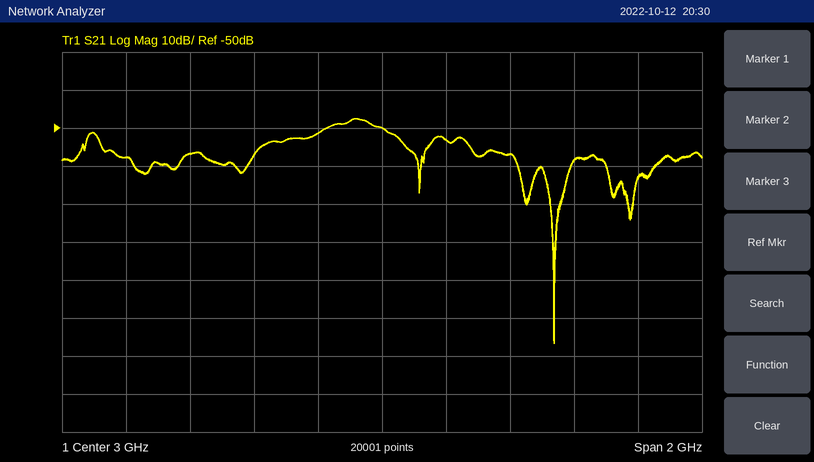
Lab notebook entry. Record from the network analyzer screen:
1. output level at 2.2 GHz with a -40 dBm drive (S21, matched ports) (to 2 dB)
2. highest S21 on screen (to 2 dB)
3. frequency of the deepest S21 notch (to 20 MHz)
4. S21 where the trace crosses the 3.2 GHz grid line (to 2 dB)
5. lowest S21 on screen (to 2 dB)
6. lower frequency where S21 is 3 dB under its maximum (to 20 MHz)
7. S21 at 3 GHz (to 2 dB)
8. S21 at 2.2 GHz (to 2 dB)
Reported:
-98 dBm
-48 dB
3.54 GHz
-54 dB
-106 dB
2.82 GHz
-50 dB
-58 dB
